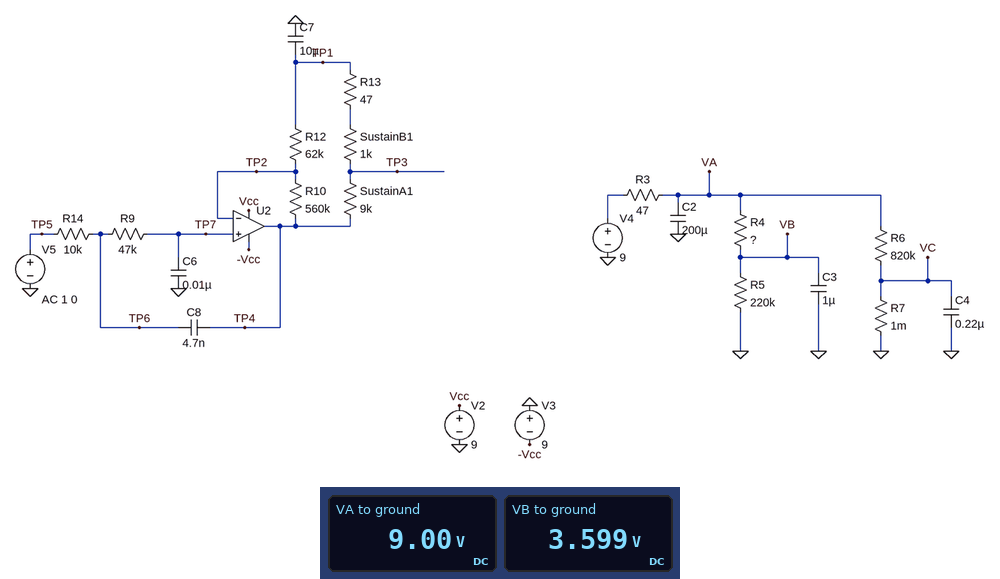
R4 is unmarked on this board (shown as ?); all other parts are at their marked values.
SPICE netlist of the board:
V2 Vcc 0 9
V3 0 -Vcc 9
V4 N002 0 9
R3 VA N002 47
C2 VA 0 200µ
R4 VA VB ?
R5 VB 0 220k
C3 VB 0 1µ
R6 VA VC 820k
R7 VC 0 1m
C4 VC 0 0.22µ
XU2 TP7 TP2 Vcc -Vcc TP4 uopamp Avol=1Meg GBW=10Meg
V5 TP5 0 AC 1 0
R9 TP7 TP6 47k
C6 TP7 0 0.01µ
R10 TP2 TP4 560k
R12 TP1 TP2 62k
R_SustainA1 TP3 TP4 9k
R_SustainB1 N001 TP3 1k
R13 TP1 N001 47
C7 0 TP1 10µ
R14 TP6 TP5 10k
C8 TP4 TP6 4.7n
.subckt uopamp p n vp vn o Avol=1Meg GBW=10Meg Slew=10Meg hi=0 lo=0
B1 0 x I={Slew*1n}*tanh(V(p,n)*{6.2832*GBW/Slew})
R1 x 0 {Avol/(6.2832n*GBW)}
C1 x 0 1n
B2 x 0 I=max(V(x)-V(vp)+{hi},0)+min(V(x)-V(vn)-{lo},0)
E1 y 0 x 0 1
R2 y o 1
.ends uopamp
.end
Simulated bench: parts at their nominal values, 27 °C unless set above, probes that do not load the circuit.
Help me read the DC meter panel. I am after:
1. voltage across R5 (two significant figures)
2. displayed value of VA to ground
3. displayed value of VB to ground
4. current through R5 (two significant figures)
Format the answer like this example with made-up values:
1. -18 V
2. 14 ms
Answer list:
1. 3.6 V
2. 9.00 V
3. 3.599 V
4. 16 µA
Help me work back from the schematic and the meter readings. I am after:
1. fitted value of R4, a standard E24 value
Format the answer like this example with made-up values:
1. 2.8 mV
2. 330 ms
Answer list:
1. 330 kΩ
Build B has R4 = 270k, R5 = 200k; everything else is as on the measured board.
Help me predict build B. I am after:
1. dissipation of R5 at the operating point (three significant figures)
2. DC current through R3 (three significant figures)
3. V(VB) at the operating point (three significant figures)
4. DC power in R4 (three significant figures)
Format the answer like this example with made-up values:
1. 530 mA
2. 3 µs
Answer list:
1. 73.3 µW
2. 30.1 µA
3. 3.83 V
4. 99.0 µW
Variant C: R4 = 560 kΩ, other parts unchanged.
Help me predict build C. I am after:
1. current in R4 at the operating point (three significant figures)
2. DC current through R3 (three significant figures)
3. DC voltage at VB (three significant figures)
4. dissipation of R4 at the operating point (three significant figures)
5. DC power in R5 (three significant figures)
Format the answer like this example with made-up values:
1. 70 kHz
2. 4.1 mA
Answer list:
1. 11.5 µA
2. 22.5 µA
3. 2.54 V
4. 74.5 µW
5. 29.3 µW
